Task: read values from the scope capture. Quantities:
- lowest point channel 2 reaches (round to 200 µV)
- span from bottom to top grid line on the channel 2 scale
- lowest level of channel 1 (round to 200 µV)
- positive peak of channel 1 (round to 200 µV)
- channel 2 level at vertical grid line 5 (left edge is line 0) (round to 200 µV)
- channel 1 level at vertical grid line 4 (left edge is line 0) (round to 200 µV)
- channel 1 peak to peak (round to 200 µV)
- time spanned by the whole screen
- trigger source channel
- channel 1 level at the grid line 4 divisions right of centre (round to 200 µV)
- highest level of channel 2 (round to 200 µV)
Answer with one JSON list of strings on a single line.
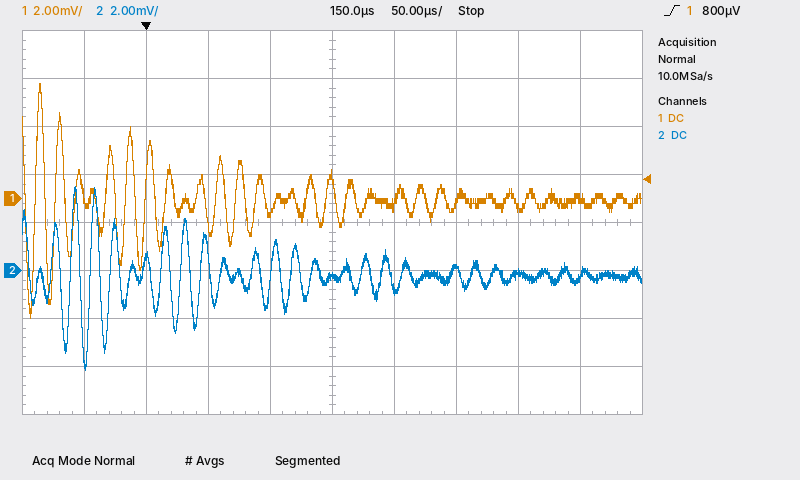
["-4.2 mV", "16 mV", "-5.0 mV", "4.8 mV", "-200 µV", "-600 µV", "9.8 mV", "500 µs", "channel 1", "0.0 mV", "3.6 mV"]
